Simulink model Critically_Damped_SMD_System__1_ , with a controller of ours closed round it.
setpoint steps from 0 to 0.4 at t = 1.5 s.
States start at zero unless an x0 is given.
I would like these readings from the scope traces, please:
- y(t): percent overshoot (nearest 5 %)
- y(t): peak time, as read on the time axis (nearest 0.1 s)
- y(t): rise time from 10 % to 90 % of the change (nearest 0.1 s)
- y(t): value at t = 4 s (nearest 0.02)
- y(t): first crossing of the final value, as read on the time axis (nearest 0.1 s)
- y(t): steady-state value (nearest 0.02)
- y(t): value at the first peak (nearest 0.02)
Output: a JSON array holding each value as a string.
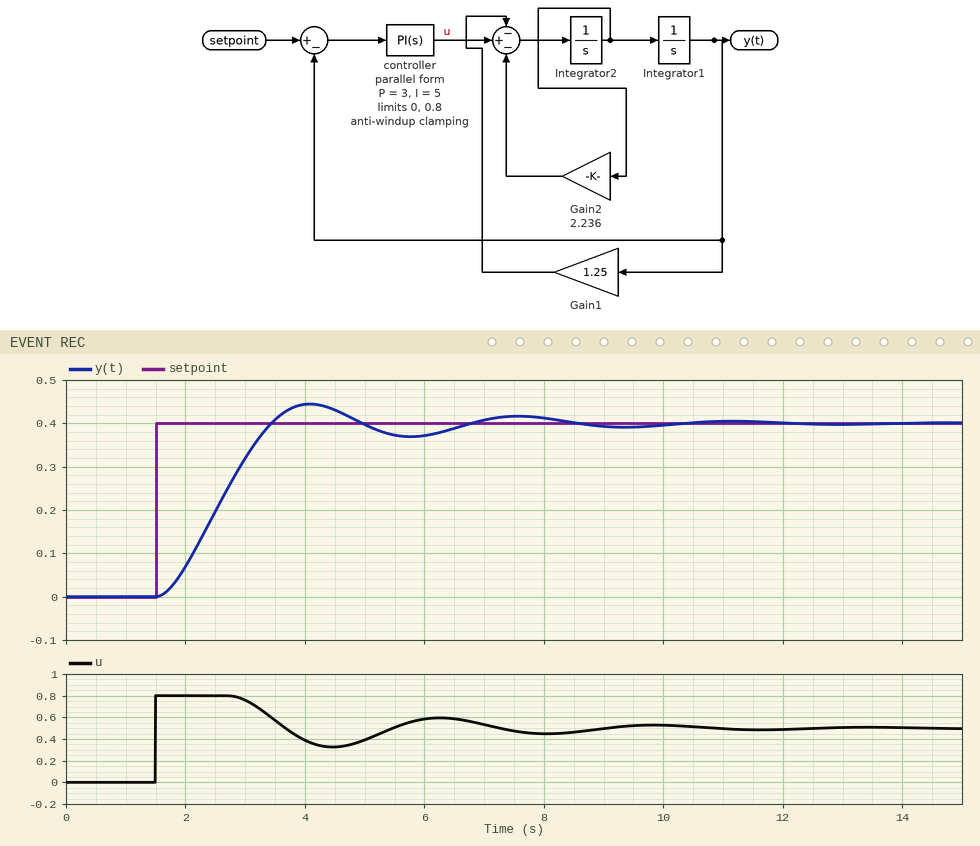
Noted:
["10 %", "4.1 s", "1.3 s", "0.44", "3.4 s", "0.40", "0.44"]
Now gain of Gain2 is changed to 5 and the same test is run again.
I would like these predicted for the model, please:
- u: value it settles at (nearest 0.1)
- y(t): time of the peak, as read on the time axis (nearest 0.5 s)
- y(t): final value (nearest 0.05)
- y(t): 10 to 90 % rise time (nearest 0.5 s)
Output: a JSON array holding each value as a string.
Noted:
["0.5", "6.5 s", "0.40", "3.0 s"]
